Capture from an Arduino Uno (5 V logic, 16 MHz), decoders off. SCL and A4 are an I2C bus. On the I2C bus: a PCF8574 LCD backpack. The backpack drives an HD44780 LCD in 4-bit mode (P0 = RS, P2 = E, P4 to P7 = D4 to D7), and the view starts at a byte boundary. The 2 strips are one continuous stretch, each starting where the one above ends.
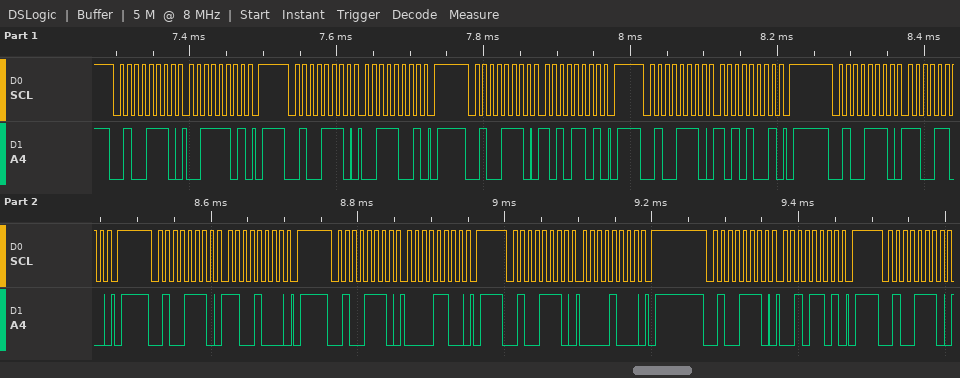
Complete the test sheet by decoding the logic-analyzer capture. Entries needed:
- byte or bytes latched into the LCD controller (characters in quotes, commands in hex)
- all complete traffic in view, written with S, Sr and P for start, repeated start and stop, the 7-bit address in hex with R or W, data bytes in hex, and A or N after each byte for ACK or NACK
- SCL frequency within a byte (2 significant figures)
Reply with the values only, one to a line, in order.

':' 0xC0
S 27W A 3D A P S 27W A 39 A P S 27W A AD A P S 27W A A9 A P S 27W A CC A P S 27W A C8 A P S 27W A 0C A P S 27W A 08 A P S 27W A 2D A P S 27W A
100 kHz
